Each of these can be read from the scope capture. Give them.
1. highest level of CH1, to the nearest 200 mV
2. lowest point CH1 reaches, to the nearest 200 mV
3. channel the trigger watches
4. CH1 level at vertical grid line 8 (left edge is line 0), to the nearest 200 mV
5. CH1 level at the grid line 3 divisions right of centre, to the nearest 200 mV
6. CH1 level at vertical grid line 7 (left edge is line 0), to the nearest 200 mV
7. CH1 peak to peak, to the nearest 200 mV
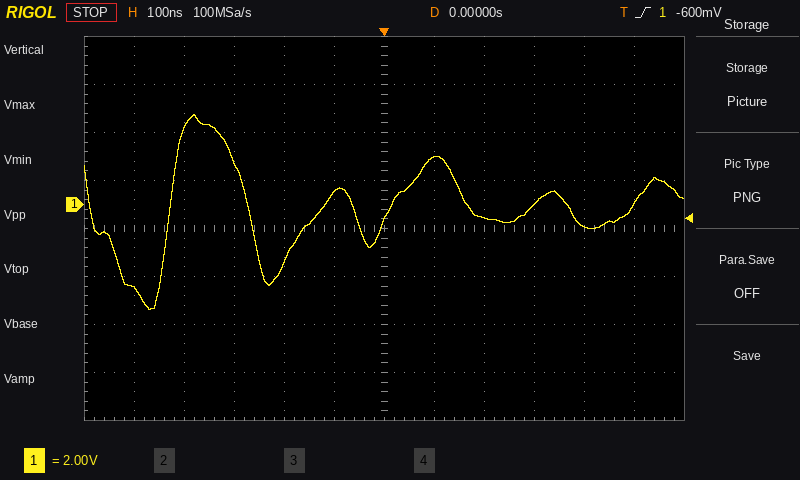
3.8 V
-4.4 V
CH1
-600 mV
0.0 V
2.0 V
8.2 V
